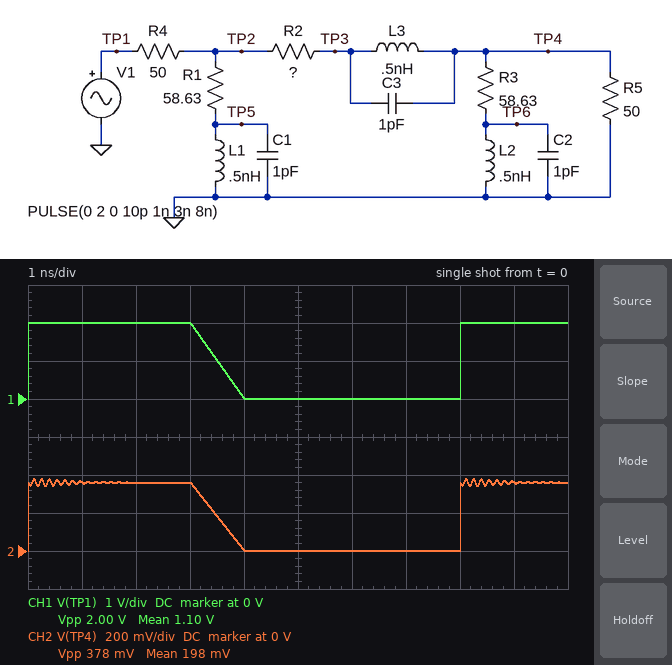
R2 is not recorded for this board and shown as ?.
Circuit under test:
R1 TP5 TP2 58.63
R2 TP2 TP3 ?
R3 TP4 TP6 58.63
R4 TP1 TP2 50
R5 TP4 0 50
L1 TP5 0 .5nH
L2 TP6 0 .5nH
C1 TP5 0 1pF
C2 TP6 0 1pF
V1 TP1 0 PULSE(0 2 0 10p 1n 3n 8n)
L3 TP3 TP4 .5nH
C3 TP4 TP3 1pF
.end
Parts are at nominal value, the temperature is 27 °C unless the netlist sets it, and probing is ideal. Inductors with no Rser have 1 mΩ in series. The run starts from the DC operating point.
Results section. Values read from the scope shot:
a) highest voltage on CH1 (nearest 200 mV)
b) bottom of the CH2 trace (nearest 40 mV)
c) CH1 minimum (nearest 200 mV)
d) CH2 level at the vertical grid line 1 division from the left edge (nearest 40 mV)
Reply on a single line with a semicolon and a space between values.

2.0 V; 0 V; 0 V; 360 mV
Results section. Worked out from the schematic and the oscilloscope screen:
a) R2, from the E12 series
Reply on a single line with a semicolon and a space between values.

27 Ω
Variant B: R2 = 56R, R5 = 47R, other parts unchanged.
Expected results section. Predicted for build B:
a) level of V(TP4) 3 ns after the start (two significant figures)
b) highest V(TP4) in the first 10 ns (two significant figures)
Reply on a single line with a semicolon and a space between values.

260 mV; 270 mV
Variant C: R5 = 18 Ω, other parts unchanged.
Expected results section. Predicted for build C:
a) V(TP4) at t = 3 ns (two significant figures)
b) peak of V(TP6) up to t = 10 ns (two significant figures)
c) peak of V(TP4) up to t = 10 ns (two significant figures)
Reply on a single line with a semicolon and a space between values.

220 mV; 57 mV; 240 mV
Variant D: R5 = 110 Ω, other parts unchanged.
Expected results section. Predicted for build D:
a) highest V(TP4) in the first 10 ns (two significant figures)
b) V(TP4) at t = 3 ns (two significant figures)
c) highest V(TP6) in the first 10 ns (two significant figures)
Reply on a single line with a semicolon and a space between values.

470 mV; 450 mV; 130 mV
